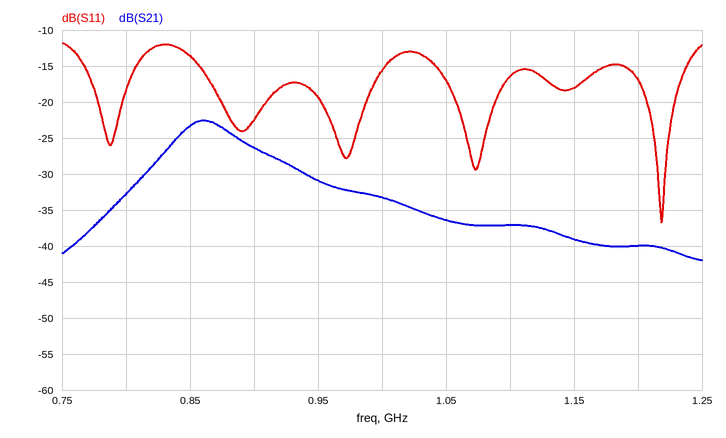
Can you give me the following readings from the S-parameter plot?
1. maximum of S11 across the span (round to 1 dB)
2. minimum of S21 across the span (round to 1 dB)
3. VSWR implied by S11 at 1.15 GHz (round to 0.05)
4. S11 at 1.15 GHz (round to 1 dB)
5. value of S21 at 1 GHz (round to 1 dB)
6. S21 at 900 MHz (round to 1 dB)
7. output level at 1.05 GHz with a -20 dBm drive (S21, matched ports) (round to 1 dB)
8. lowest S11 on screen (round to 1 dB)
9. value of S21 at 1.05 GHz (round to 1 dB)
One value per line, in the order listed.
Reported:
-12 dB
-42 dB
1.30
-18 dB
-33 dB
-26 dB
-56 dBm
-37 dB
-36 dB
